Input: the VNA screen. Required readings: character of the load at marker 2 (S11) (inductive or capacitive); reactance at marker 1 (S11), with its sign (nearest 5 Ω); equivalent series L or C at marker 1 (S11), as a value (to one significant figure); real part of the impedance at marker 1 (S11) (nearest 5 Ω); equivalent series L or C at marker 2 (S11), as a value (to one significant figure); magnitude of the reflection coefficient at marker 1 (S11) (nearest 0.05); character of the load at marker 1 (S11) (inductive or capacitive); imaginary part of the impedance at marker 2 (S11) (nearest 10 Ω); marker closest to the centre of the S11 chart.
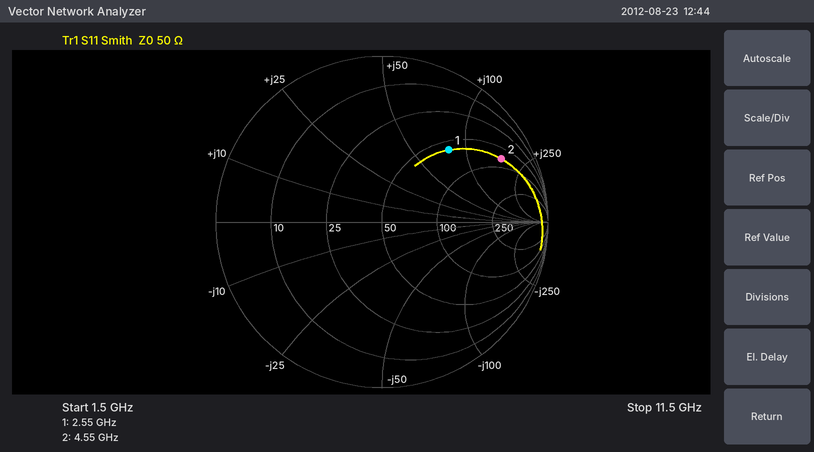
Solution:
inductive
+80 Ω
5 nH
60 Ω
6 nH
0.60
inductive
+170 Ω
marker 1
